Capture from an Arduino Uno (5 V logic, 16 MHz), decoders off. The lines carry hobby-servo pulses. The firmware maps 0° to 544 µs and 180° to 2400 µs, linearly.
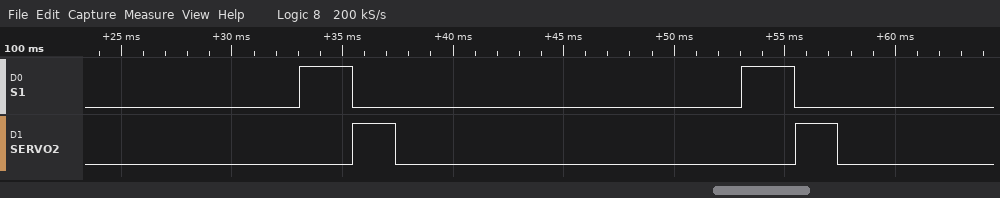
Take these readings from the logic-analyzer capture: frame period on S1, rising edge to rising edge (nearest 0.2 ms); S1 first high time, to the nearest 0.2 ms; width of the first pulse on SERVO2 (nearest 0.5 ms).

20.0 ms
2.4 ms
2.0 ms
